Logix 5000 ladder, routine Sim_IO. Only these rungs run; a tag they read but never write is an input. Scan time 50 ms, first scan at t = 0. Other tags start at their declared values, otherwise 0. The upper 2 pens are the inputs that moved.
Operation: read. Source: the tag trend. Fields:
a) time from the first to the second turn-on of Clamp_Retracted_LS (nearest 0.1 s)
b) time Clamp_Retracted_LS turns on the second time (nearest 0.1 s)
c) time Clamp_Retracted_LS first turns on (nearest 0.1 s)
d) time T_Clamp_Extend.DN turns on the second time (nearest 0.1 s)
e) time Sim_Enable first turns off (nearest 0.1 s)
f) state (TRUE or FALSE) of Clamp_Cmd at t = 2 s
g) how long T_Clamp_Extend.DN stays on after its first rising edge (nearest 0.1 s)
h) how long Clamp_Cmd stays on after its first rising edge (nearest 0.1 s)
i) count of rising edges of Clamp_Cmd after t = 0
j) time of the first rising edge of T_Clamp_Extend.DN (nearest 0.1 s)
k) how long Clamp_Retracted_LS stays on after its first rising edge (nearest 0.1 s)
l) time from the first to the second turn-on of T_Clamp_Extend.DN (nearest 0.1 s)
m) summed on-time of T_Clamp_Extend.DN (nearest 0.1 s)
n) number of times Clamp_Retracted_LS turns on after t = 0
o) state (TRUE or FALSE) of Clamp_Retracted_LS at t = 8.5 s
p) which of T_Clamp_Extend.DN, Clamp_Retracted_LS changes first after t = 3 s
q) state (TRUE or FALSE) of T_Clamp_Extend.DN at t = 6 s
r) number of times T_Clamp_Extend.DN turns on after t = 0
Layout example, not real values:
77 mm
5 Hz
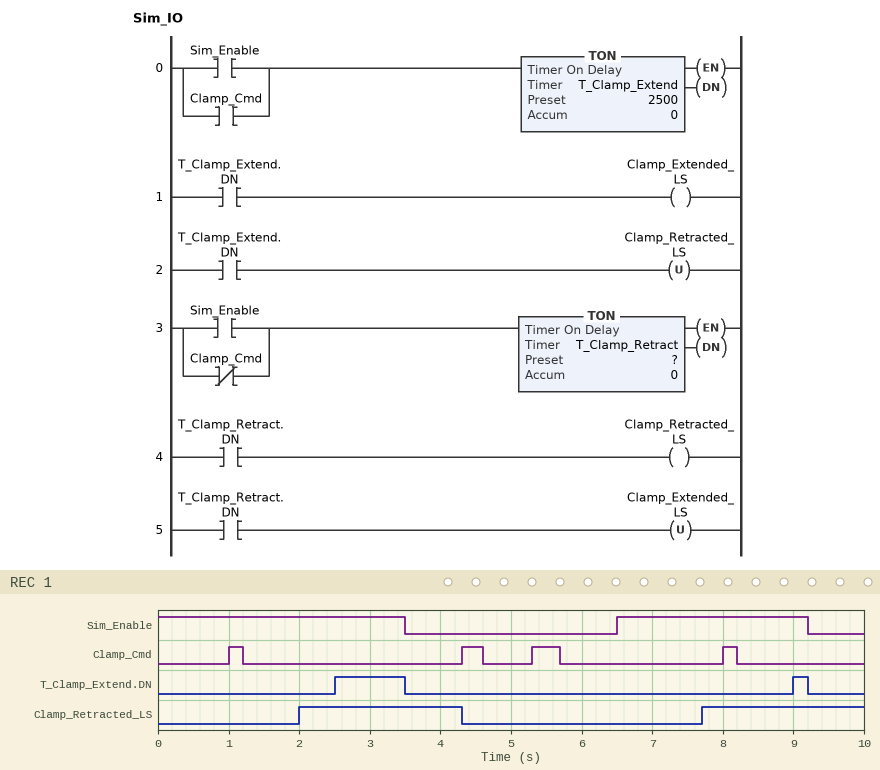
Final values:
5.7 s
7.7 s
2.0 s
9.0 s
3.5 s
FALSE
1.0 s
0.2 s
4
2.5 s
2.3 s
6.5 s
1.2 s
2
TRUE
T_Clamp_Extend.DN
FALSE
2
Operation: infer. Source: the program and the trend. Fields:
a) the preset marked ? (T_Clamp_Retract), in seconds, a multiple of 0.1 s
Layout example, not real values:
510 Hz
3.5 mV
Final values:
2.0 s
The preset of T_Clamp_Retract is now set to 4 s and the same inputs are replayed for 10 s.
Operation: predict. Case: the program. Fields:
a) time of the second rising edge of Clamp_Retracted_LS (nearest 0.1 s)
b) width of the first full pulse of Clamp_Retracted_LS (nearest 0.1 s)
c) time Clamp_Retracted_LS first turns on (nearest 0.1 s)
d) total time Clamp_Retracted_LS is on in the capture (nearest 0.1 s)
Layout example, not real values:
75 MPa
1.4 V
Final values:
9.7 s
0.3 s
4.0 s
0.6 s
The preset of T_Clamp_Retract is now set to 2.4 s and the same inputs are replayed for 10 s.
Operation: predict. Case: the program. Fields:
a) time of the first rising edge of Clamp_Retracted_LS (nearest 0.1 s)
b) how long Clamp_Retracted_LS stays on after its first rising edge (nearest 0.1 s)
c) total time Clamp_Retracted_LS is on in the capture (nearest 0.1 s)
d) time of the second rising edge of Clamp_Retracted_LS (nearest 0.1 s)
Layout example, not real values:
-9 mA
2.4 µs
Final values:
2.4 s
1.9 s
3.8 s
8.1 s
